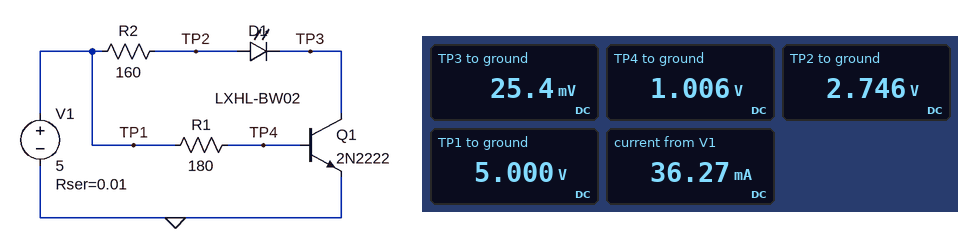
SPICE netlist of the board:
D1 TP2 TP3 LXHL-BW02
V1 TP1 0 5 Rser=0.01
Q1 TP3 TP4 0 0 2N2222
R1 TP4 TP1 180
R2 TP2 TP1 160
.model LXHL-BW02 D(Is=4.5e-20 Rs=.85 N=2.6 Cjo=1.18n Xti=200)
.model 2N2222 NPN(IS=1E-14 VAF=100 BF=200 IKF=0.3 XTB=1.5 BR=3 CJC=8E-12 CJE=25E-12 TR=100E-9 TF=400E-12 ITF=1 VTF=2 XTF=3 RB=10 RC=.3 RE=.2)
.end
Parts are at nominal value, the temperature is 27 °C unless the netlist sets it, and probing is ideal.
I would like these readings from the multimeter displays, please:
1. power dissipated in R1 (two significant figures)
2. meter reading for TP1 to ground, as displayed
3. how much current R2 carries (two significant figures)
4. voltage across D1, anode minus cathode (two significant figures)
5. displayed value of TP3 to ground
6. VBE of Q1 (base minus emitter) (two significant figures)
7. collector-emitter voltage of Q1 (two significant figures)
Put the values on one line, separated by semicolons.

89 mW; 5.000 V; 14 mA; 2.7 V; 25.4 mV; 1.0 V; 25 mV
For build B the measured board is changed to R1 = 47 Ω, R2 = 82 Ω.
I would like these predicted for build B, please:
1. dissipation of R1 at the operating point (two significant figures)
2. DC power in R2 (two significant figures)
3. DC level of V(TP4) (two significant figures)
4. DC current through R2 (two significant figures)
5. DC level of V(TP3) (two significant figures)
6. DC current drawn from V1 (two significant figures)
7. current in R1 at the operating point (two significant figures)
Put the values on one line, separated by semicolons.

250 mW; 58 mW; 1.6 V; 27 mA; 43 mV; 100 mA; 73 mA
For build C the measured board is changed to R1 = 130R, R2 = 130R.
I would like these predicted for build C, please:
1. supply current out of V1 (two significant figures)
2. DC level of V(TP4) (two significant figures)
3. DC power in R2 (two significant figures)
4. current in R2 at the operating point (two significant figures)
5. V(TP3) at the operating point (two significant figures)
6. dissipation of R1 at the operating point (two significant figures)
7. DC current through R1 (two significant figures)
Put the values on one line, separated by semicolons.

47 mA; 1.1 V; 38 mW; 17 mA; 29 mV; 120 mW; 30 mA
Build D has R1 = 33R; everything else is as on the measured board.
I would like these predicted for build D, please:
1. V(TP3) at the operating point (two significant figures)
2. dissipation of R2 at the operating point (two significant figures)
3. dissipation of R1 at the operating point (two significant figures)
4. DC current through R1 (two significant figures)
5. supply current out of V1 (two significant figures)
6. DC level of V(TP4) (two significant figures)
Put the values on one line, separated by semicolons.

40 mV; 31 mW; 310 mW; 97 mA; 110 mA; 1.8 V
